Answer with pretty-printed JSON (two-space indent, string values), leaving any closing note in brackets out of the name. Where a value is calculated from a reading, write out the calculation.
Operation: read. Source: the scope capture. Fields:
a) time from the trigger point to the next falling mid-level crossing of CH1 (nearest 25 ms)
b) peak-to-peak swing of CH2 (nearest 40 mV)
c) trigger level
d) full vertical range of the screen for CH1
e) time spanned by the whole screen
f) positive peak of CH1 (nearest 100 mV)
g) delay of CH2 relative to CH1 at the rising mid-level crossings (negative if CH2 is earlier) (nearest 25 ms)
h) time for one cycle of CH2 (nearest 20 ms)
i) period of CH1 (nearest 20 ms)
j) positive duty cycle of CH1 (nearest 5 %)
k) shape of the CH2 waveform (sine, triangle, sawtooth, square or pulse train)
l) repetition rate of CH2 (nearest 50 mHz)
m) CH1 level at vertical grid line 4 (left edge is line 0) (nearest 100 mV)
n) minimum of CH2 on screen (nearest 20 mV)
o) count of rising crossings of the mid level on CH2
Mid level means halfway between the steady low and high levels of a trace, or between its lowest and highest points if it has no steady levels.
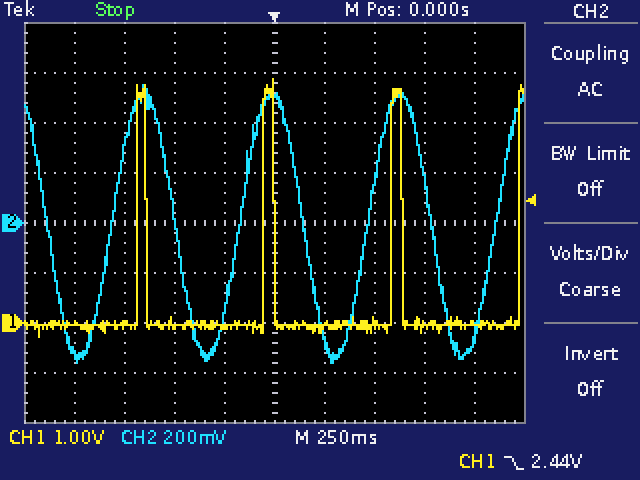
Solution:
{
  "time from the trigger point to the next falling mid-level crossing of CH1": "650 ms",
  "peak-to-peak swing of CH2": "1.12 V",
  "trigger level": "2.44 V",
  "full vertical range of the screen for CH1": "8 V",
  "time spanned by the whole screen": "2.5 s",
  "positive peak of CH1": "4.9 V",
  "delay of CH2 relative to CH1 at the rising mid-level crossings (negative if CH2 is earlier)": "-125 ms",
  "time for one cycle of CH2": "640 ms",
  "period of CH1": "640 ms",
  "positive duty cycle of CH1": "10 %",
  "shape of the CH2 waveform": "sine",
  "repetition rate of CH2": "1 / 640 ms ≈ 1.56 Hz, so 1.55 Hz to the nearest 50 mHz",
  "CH1 level at vertical grid line 4 (left edge is line 0)": "-100 mV",
  "minimum of CH2 on screen": "-560 mV",
  "count of rising crossings of the mid level on CH2": "4"
}
